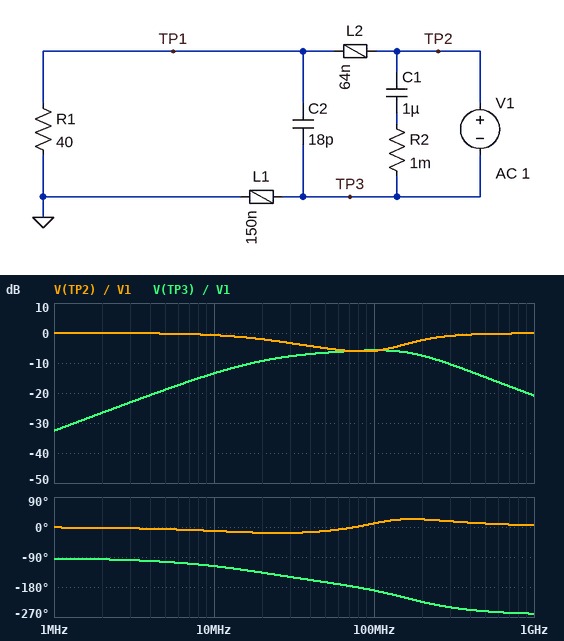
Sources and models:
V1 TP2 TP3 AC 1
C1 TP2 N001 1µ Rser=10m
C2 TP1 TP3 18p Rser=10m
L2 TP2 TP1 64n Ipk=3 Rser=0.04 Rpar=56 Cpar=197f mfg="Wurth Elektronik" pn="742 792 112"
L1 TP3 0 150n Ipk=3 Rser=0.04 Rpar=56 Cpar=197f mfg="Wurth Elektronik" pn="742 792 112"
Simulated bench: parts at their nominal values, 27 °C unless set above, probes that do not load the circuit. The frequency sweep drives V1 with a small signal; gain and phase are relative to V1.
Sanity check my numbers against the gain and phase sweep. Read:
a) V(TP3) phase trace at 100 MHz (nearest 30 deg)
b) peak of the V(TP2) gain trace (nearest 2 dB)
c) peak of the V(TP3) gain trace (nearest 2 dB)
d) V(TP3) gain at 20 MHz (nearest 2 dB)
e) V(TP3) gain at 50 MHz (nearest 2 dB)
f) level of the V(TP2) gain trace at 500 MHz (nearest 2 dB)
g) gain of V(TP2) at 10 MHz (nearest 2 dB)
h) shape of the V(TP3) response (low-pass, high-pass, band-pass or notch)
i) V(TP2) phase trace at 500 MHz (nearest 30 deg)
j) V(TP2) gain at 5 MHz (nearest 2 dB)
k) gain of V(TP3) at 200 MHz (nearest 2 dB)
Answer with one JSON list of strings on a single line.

["-180 deg", "0 dB", "-6 dB", "-10 dB", "-6 dB", "0 dB", "0 dB", "band-pass", "0 deg", "0 dB", "-8 dB"]
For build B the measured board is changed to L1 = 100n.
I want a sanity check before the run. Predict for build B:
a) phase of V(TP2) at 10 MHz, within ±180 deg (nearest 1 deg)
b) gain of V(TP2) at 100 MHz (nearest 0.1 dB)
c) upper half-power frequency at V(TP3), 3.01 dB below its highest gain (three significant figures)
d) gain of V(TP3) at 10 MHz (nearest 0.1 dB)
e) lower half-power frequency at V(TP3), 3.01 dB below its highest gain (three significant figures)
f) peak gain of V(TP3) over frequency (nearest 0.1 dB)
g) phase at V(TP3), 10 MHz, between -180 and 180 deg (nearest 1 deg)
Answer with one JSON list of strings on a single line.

["-8 deg", "-5.6 dB", "262 MHz", "-16.6 dB", "32.1 MHz", "-6.3 dB", "-111 deg"]
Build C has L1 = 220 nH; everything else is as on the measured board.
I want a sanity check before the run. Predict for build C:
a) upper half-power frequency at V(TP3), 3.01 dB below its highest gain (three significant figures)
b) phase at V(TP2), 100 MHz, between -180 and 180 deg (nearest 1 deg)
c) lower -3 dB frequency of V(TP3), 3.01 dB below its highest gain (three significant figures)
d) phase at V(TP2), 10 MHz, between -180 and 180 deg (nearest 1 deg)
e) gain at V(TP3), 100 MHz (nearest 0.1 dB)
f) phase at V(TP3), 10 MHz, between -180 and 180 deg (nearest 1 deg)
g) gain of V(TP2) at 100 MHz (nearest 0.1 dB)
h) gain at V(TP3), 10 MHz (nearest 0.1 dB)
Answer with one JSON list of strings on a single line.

["229 MHz", "17 deg", "16.0 MHz", "-16 deg", "-5.4 dB", "-125 deg", "-5.9 dB", "-10.8 dB"]
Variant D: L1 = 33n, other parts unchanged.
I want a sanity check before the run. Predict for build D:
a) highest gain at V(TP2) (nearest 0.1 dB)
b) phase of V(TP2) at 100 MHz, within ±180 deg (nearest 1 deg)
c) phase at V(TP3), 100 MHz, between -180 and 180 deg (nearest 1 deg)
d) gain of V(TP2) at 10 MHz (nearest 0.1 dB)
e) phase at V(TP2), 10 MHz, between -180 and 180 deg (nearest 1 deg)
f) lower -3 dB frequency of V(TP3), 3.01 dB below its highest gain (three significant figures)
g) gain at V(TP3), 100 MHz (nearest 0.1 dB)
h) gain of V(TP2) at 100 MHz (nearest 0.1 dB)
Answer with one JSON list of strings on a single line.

["0 dB", "-9 deg", "-156 deg", "-0.1 dB", "-3 deg", "74.0 MHz", "-11.0 dB", "-2.5 dB"]
